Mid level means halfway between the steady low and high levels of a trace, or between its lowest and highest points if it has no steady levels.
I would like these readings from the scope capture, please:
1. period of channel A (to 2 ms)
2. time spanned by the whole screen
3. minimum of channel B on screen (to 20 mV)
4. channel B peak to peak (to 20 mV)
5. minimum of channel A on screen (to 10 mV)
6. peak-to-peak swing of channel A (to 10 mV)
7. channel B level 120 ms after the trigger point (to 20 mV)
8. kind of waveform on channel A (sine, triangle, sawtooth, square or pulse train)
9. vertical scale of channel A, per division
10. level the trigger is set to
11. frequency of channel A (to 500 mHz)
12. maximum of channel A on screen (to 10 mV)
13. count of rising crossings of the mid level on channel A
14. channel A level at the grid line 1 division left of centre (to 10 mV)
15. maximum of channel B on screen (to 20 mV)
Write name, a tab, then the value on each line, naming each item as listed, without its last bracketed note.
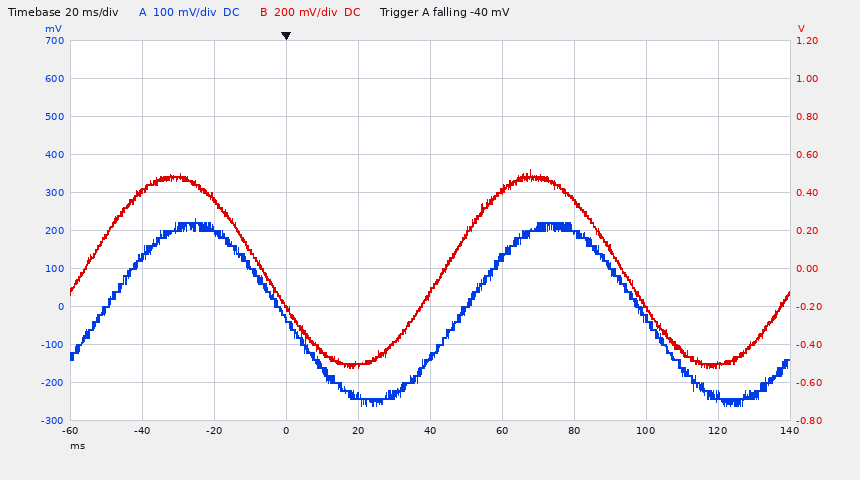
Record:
period of channel A	100 ms
time spanned by the whole screen	200 ms
minimum of channel B on screen	-520 mV
channel B peak to peak	1.04 V
minimum of channel A on screen	-260 mV
peak-to-peak swing of channel A	490 mV
channel B level 120 ms after the trigger point	-500 mV
kind of waveform on channel A	sine
vertical scale of channel A, per division	100 mV
level the trigger is set to	-40 mV
frequency of channel A	10.0 Hz
maximum of channel A on screen	230 mV
count of rising crossings of the mid level on channel A	2
channel A level at the grid line 1 division left of centre	-230 mV
maximum of channel B on screen	520 mV
